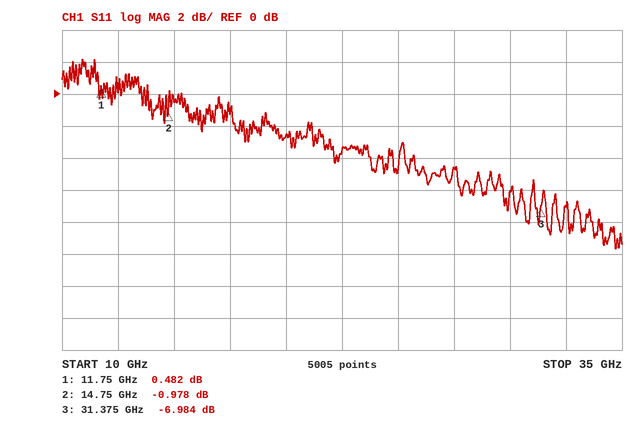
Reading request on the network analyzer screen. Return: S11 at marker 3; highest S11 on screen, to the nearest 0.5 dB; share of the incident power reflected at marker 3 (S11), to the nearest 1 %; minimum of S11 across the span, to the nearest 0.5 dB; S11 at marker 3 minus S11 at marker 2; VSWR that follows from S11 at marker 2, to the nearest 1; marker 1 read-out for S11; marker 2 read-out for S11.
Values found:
-6.984 dB
2.0 dB
20 %
-9.5 dB
-6.006 dB
18
0.482 dB
-0.978 dB
